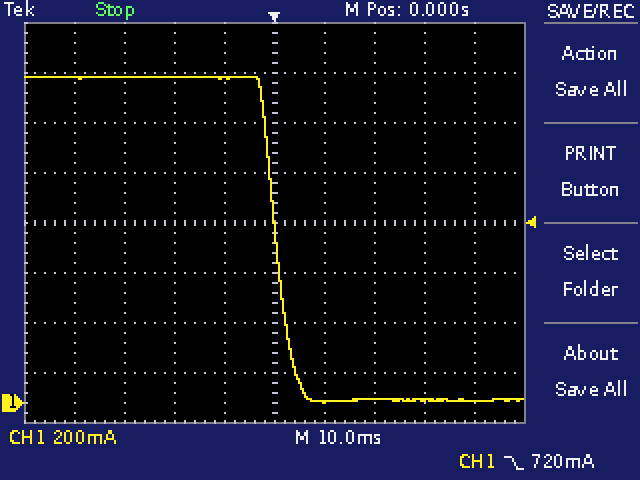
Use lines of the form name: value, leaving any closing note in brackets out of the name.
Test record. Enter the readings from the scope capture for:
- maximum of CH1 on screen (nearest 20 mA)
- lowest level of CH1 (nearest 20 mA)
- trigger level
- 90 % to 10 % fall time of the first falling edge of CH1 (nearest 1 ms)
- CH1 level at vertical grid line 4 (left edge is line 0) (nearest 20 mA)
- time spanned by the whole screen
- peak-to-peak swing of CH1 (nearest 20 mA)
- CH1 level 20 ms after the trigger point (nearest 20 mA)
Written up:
maximum of CH1 on screen: 1.30 A
lowest level of CH1: 0 mA
trigger level: 720 mA
90 % to 10 % fall time of the first falling edge of CH1: 6 ms
CH1 level at vertical grid line 4 (left edge is line 0): 1.30 A
time spanned by the whole screen: 100 ms
peak-to-peak swing of CH1: 1.30 A
CH1 level 20 ms after the trigger point: 20 mA
